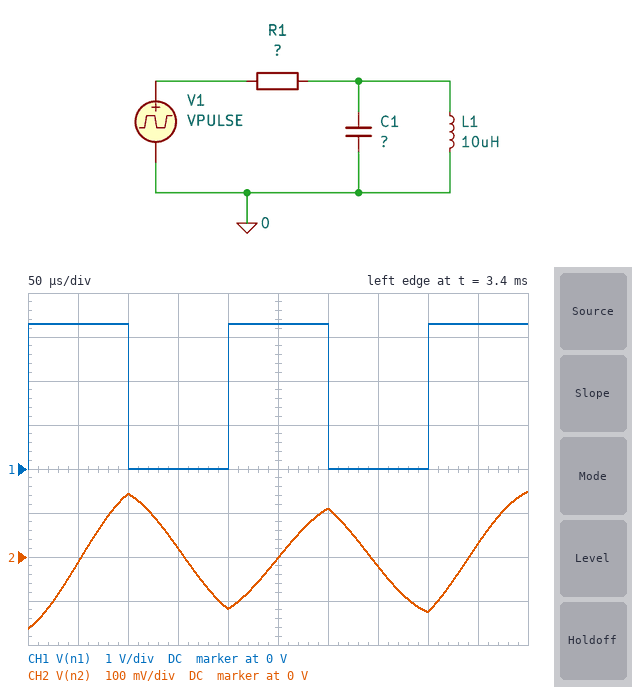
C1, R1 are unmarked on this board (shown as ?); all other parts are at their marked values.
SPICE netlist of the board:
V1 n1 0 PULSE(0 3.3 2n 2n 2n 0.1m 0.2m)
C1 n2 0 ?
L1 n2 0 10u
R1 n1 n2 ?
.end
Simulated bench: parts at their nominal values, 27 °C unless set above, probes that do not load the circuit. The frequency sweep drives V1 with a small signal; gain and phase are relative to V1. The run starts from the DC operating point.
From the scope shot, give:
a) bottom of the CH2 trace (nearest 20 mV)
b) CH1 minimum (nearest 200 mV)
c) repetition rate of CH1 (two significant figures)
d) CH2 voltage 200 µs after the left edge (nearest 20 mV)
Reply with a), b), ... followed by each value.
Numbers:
a) -160 mV
b) 0 V
c) 5.0 kHz
d) -120 mV
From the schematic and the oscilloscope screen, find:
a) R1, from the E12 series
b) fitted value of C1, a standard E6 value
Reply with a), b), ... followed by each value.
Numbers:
a) 4.7 Ω
b) 220 µF
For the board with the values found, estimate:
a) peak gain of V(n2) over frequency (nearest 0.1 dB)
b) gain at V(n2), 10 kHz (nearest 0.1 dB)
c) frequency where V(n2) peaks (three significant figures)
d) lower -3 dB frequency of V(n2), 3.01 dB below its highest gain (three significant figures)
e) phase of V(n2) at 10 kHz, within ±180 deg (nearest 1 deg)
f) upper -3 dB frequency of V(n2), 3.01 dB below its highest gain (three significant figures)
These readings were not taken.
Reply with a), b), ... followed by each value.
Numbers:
a) 0 dB
b) -35.2 dB
c) 3.39 kHz
d) 3.32 kHz
e) -89 deg
f) 3.47 kHz
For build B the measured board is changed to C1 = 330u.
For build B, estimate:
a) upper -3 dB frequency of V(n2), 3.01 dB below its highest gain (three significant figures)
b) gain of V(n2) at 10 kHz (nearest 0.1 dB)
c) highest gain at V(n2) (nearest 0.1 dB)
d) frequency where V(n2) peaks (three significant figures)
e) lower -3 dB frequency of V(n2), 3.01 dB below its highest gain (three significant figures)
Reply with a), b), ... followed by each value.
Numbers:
a) 2.82 kHz
b) -39.1 dB
c) 0 dB
d) 2.77 kHz
e) 2.72 kHz
